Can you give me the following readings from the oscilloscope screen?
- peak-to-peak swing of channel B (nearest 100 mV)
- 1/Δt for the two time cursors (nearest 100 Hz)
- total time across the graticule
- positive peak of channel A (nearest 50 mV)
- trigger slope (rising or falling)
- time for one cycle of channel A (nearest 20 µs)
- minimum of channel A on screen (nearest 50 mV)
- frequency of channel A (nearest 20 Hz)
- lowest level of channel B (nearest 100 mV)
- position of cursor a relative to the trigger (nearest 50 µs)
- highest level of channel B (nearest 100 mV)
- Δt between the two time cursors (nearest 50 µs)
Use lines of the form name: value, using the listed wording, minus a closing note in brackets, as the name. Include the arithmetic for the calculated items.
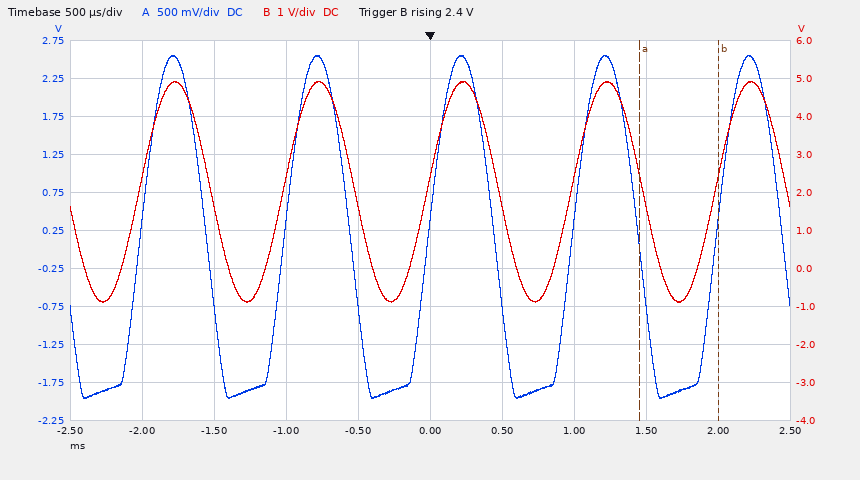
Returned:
peak-to-peak swing of channel B: 4.9 V − (-900 mV) = 5.8 V
1/Δt for the two time cursors: 1 / 550 µs ≈ 1.8 kHz
total time across the graticule: 5 ms
positive peak of channel A: 2.55 V
trigger slope: rising
time for one cycle of channel A: 1.00 ms
minimum of channel A on screen: -1.95 V
frequency of channel A: 1 / 1.00 ms ≈ 1.00 kHz
lowest level of channel B: -900 mV
position of cursor a relative to the trigger: +1.45 ms
highest level of channel B: 4.9 V
Δt between the two time cursors: 550 µs
